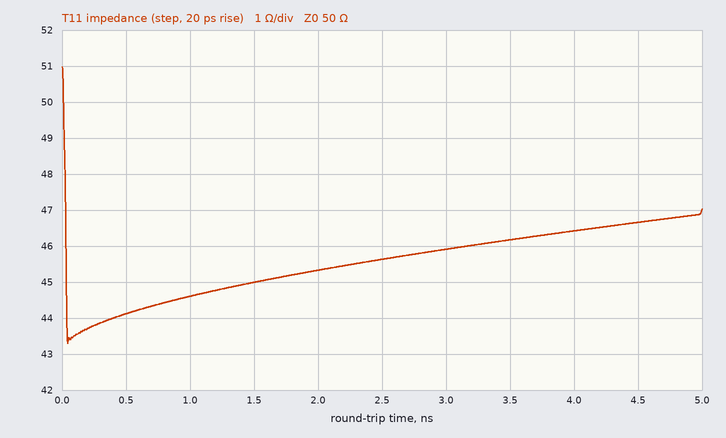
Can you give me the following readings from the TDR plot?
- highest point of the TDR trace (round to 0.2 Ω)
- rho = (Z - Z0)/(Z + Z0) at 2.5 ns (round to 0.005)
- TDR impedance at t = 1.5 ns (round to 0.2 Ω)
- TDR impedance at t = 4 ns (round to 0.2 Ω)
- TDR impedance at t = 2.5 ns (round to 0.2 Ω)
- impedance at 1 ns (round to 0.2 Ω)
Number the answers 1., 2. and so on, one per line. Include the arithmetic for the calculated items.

1. 51.0 Ω
2. (45.6 − 50)/(45.6 + 50) ≈ -0.0460, so -0.045 to the nearest 0.005
3. 45.0 Ω
4. 46.4 Ω
5. 45.6 Ω
6. 44.6 Ω
